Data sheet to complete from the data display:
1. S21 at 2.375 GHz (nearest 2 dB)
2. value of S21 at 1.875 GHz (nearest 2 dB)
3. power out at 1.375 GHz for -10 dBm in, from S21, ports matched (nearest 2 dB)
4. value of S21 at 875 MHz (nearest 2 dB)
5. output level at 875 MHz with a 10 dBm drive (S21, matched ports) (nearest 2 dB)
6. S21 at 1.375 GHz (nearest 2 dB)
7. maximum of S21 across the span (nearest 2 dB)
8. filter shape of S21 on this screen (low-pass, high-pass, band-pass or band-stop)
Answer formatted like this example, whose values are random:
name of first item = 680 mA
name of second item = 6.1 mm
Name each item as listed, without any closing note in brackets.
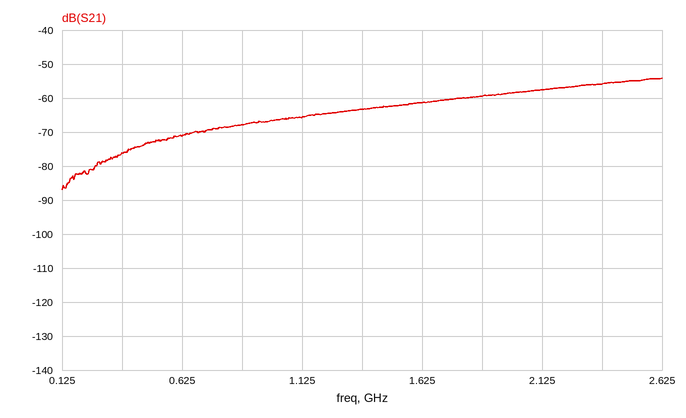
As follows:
S21 at 2.375 GHz = -56 dB
value of S21 at 1.875 GHz = -60 dB
power out at 1.375 GHz for -10 dBm in, from S21, ports matched = -74 dBm
value of S21 at 875 MHz = -68 dB
output level at 875 MHz with a 10 dBm drive (S21, matched ports) = -58 dBm
S21 at 1.375 GHz = -64 dB
maximum of S21 across the span = -54 dB
filter shape of S21 on this screen = high-pass
